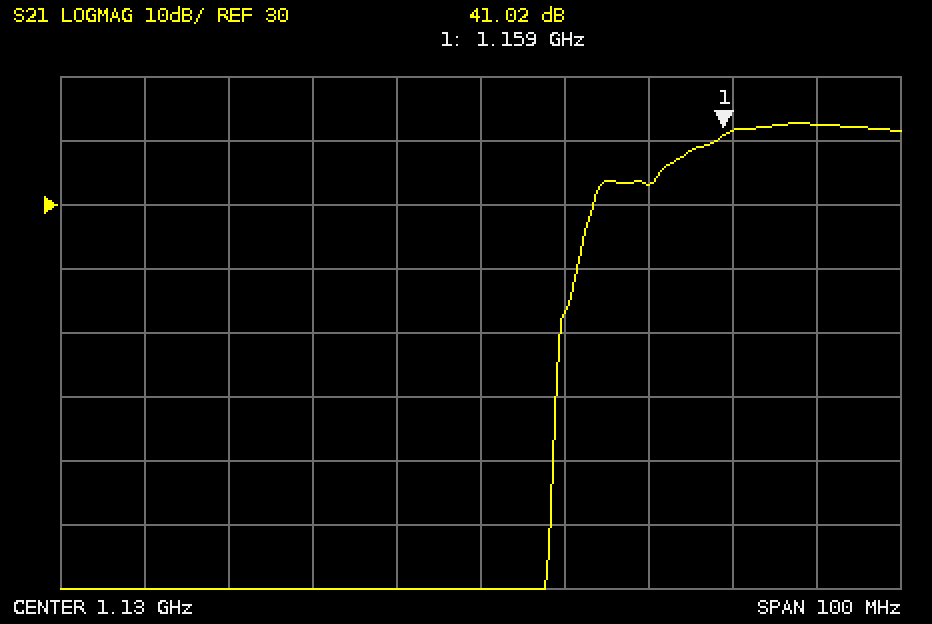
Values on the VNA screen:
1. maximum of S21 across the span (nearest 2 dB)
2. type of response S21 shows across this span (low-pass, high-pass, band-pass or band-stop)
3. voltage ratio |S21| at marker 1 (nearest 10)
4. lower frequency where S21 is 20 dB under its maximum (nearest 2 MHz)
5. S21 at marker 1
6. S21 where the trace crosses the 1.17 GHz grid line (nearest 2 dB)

42 dB
high-pass
110
1.142 GHz
41.02 dB
42 dB
